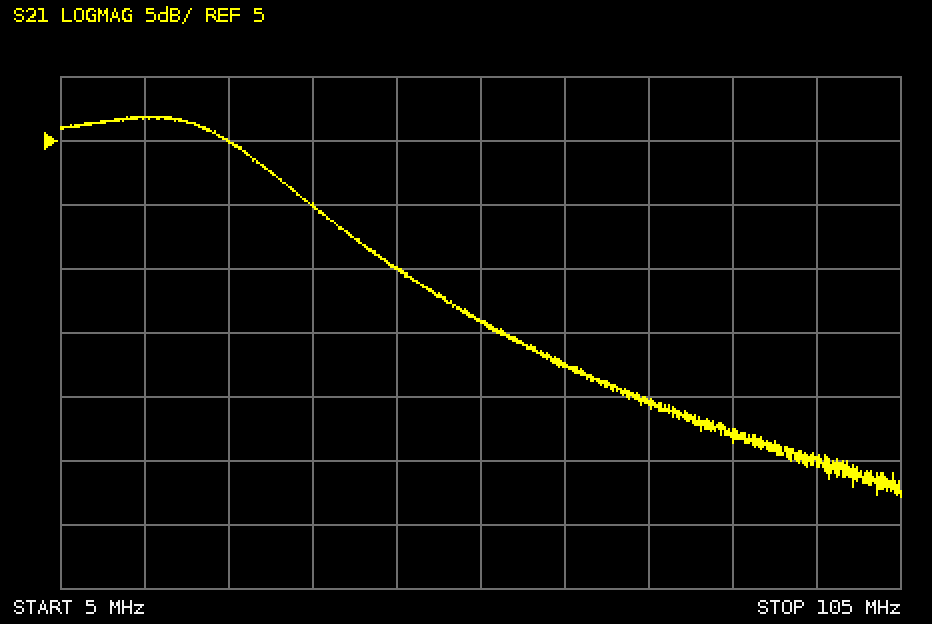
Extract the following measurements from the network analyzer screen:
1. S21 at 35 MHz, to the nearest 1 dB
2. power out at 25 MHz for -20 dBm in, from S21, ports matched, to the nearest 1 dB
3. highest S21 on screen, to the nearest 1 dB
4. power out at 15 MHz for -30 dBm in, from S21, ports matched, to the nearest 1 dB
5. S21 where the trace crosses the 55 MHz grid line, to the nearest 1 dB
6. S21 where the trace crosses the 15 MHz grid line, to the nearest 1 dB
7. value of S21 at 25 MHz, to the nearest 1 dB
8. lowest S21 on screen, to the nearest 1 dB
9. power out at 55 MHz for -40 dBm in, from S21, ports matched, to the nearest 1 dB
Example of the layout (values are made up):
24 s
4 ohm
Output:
0 dB
-15 dBm
7 dB
-23 dBm
-9 dB
7 dB
5 dB
-23 dB
-49 dBm
